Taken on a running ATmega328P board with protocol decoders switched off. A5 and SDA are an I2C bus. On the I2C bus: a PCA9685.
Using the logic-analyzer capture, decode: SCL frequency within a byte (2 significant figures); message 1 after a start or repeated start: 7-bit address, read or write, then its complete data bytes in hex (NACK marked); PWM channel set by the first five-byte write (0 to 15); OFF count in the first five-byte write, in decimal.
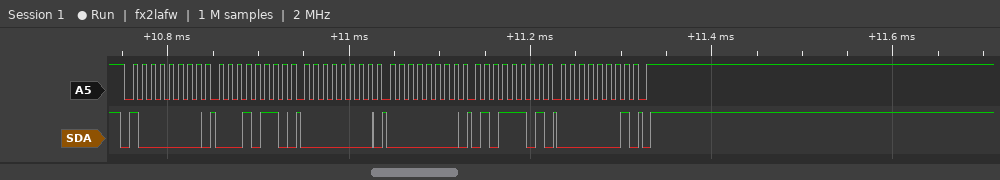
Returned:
100 kHz
0x40 write: 16 00 00 5D 01
4
349
